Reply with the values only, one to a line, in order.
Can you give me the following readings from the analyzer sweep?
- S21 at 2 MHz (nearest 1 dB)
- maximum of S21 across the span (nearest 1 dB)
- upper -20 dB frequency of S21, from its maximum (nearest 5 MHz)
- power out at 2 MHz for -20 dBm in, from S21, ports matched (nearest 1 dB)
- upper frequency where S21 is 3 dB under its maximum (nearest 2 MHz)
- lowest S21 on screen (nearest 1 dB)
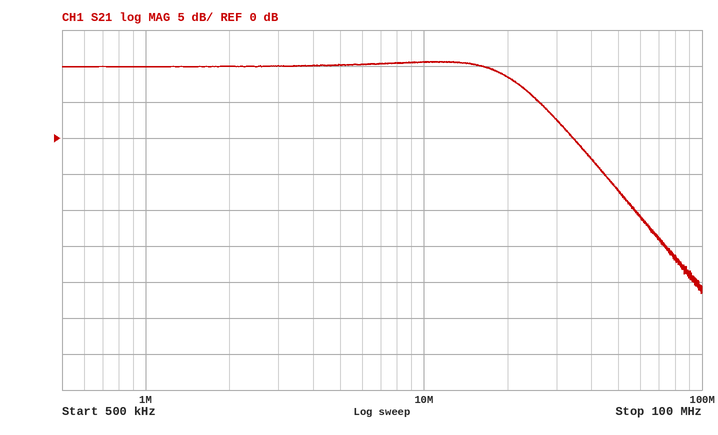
10 dB
11 dB
55 MHz
-10 dBm
22 MHz
-22 dB
